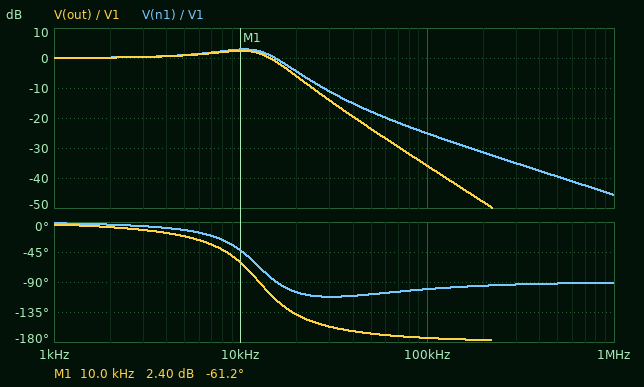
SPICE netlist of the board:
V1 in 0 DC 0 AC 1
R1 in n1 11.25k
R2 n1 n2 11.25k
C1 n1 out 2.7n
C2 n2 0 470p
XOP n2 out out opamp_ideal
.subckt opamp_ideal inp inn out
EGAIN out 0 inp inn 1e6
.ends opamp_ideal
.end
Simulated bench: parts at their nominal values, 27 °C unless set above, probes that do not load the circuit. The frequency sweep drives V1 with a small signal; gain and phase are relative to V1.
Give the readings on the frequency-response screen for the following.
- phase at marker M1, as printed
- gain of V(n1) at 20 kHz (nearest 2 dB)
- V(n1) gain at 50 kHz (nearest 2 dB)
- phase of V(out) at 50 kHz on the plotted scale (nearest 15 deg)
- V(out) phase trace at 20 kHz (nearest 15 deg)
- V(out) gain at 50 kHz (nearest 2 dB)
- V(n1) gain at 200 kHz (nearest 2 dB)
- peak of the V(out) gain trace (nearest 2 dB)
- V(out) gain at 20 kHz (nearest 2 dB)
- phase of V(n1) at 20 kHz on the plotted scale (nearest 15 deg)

-61.2 deg
-4 dB
-18 dB
-165 deg
-135 deg
-24 dB
-32 dB
2 dB
-6 dB
-105 deg
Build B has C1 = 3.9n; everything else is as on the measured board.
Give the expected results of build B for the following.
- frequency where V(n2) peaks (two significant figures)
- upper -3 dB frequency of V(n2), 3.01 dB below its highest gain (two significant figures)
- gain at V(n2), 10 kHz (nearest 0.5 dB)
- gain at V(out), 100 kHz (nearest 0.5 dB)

9.1 kHz
12 kHz
3.5 dB
-39.0 dB
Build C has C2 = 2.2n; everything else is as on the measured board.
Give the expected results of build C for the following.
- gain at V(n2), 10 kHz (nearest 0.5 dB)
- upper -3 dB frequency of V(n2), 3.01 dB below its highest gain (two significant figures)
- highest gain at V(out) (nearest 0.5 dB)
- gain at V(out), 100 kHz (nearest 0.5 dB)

-11.5 dB
4.3 kHz
0 dB
-49.5 dB
